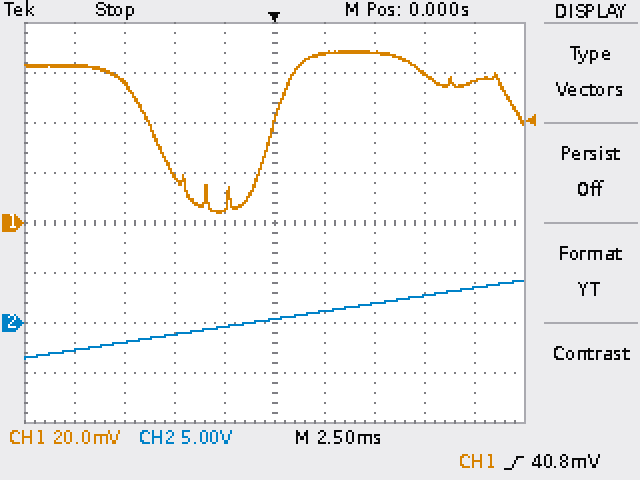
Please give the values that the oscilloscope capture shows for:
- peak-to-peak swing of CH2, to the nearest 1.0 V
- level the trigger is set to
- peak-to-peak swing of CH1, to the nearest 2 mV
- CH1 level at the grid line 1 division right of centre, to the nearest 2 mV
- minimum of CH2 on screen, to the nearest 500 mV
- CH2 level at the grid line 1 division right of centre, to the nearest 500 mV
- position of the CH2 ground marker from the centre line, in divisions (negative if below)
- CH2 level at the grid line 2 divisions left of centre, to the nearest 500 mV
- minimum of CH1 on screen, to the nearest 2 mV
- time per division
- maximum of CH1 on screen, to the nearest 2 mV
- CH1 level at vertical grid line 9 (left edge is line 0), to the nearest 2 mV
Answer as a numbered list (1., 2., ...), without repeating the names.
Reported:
1. 8.0 V
2. 40.8 mV
3. 64 mV
4. 68 mV
5. -3.5 V
6. 1.0 V
7. -2.0 div
8. -1.0 V
9. 4 mV
10. 2.5 ms
11. 68 mV
12. 56 mV
